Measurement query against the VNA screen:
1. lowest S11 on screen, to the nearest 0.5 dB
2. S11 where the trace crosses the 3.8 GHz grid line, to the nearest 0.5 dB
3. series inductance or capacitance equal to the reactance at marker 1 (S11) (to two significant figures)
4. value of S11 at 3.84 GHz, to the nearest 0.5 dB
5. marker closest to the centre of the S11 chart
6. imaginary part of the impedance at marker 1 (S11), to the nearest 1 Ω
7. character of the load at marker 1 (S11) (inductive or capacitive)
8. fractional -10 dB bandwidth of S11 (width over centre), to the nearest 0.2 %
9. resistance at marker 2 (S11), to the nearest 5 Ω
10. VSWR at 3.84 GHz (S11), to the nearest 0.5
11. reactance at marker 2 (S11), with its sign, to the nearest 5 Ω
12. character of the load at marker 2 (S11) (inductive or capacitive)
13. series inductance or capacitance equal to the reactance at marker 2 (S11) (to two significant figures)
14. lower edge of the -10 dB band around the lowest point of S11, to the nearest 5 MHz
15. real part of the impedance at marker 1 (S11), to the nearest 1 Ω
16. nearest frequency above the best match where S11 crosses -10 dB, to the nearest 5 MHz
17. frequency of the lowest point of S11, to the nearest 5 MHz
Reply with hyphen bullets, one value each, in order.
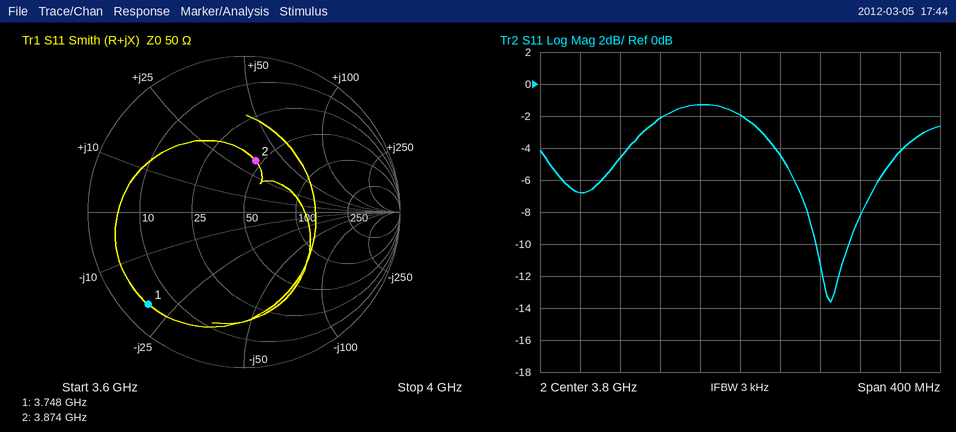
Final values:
- -13.5 dB
- -2.0 dB
- 2.1 pF
- -4.5 dB
- marker 2
- -20 Ω
- capacitive
- 0.8 %
- 45 Ω
- 4.0
- +35 Ω
- inductive
- 1.4 nH
- 3.875 GHz
- 5 Ω
- 3.910 GHz
- 3.890 GHz
